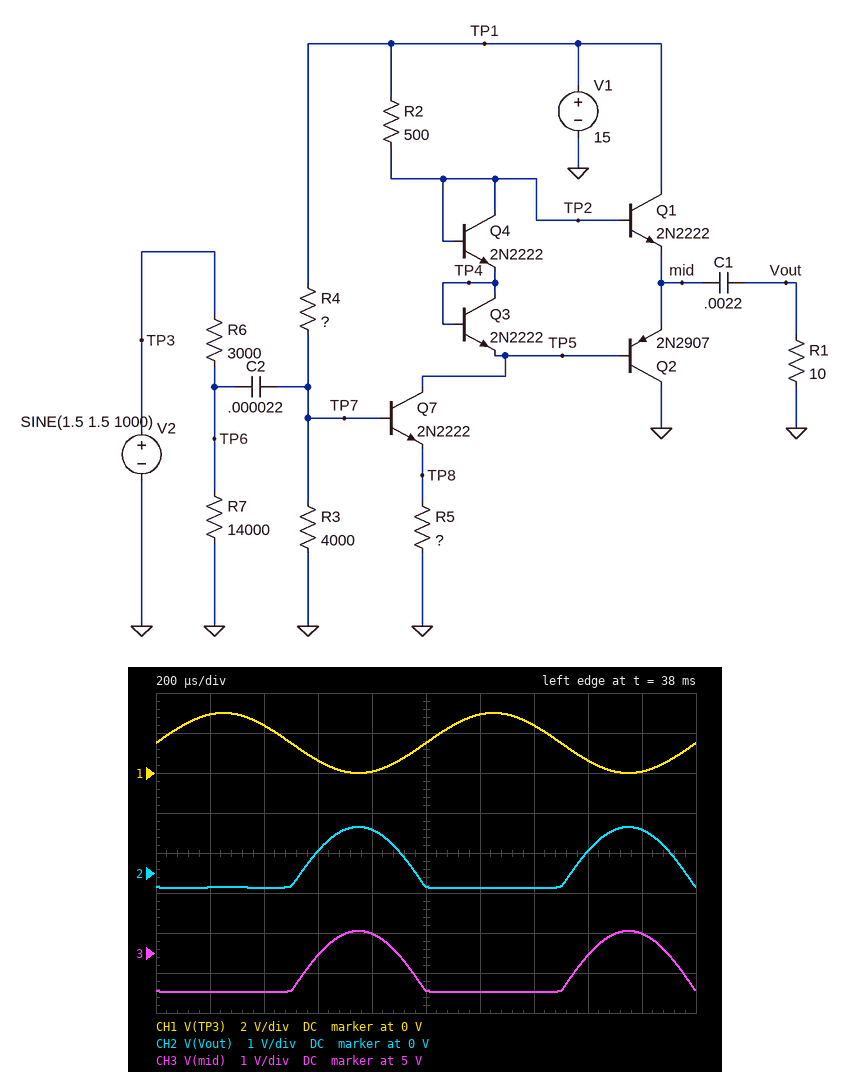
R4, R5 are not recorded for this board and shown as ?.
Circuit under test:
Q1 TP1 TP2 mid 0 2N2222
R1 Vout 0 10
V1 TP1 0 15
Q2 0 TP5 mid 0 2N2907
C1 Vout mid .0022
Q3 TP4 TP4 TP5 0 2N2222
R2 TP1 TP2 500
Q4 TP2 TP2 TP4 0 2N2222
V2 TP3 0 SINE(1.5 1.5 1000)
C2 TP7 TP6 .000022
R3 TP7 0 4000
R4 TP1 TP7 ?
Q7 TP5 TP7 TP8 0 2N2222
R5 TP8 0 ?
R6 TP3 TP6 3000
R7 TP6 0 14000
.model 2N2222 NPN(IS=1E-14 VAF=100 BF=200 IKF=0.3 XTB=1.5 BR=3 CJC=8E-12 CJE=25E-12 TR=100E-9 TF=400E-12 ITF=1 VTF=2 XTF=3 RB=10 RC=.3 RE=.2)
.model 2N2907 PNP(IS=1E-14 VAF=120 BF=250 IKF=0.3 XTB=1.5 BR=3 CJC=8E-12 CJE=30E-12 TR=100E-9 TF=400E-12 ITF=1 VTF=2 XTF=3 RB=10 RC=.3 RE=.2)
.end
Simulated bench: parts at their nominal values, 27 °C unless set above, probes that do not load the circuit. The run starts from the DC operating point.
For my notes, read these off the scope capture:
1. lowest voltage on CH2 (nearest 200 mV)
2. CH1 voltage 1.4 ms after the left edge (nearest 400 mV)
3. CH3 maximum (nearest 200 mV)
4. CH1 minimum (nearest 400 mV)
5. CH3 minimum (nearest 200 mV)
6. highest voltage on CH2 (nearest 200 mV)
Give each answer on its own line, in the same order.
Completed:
-400 mV
2.4 V
5.6 V
0 V
4.0 V
1.2 V
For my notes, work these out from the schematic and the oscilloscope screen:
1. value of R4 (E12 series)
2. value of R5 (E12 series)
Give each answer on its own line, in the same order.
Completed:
10 kΩ
150 Ω
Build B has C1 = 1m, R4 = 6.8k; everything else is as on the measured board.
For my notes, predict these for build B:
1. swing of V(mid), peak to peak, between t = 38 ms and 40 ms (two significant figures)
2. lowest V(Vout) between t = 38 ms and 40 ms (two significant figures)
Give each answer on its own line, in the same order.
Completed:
55 mV
-23 mV
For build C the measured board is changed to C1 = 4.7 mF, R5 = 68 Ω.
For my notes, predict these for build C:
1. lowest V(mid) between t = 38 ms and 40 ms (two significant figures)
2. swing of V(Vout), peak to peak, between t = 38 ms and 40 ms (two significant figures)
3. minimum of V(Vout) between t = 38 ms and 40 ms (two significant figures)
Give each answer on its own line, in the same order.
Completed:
2.5 V
19 mV
-5.3 mV
